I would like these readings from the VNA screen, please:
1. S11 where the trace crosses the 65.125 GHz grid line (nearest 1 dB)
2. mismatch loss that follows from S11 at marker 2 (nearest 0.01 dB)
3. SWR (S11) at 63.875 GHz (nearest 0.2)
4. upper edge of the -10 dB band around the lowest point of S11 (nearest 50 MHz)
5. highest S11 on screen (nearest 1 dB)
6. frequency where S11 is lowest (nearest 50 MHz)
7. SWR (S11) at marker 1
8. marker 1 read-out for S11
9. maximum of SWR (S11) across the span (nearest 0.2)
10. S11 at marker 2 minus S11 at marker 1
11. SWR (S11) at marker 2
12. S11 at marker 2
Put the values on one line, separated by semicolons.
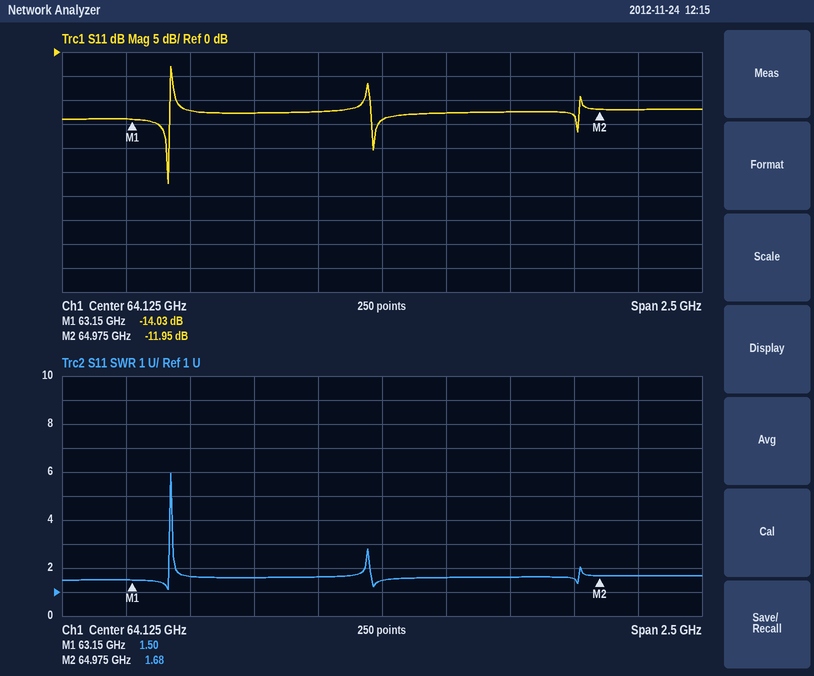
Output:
-12 dB; 0.29 dB; 1.6; 63.30 GHz; -3 dB; 63.30 GHz; 1.50; -14.03 dB; 6.0; 2.08 dB; 1.68; -11.95 dB
